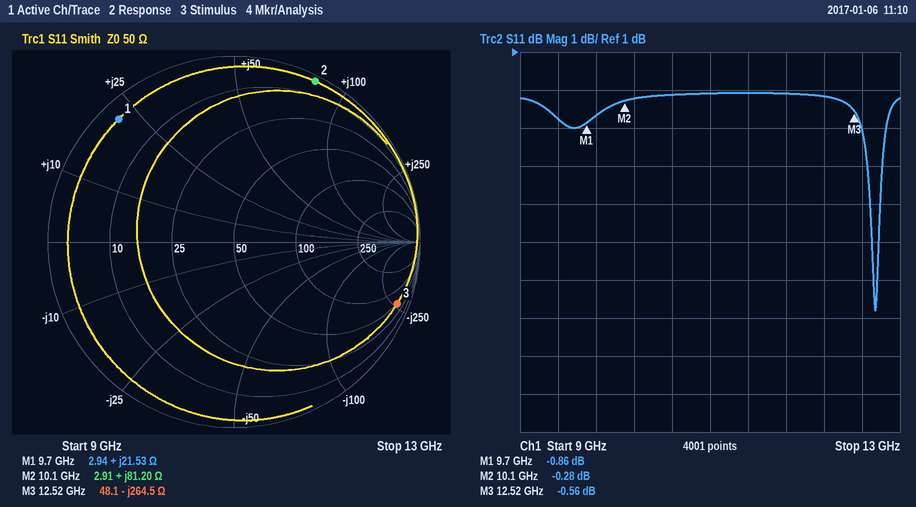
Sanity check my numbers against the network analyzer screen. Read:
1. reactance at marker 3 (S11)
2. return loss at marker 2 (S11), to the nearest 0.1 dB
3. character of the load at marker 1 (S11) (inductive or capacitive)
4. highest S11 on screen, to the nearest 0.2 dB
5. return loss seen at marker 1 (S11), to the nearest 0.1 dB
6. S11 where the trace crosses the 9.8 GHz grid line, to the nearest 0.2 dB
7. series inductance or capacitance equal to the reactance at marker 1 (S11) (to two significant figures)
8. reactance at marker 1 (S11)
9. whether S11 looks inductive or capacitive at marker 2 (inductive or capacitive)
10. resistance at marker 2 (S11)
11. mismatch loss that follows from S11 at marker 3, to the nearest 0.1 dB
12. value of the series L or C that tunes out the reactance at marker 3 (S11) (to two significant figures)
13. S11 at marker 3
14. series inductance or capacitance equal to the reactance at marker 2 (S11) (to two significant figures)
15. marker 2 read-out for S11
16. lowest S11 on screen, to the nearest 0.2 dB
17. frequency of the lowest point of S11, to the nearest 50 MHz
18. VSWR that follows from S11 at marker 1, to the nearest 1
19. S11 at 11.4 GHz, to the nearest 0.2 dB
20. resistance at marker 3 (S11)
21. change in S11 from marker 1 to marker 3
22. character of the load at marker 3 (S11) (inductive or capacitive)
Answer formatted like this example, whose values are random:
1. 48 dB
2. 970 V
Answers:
1. -264.5 Ω
2. 0.3 dB
3. inductive
4. 0.0 dB
5. 0.9 dB
6. -0.6 dB
7. 350 pH
8. +21.53 Ω
9. inductive
10. 2.91 Ω
11. 9.2 dB
12. 3.4 nH
13. -0.56 dB
14. 1.3 nH
15. -0.28 dB
16. -5.8 dB
17. 12.75 GHz
18. 20
19. 0.0 dB
20. 48.1 Ω
21. 0.30 dB
22. capacitive
